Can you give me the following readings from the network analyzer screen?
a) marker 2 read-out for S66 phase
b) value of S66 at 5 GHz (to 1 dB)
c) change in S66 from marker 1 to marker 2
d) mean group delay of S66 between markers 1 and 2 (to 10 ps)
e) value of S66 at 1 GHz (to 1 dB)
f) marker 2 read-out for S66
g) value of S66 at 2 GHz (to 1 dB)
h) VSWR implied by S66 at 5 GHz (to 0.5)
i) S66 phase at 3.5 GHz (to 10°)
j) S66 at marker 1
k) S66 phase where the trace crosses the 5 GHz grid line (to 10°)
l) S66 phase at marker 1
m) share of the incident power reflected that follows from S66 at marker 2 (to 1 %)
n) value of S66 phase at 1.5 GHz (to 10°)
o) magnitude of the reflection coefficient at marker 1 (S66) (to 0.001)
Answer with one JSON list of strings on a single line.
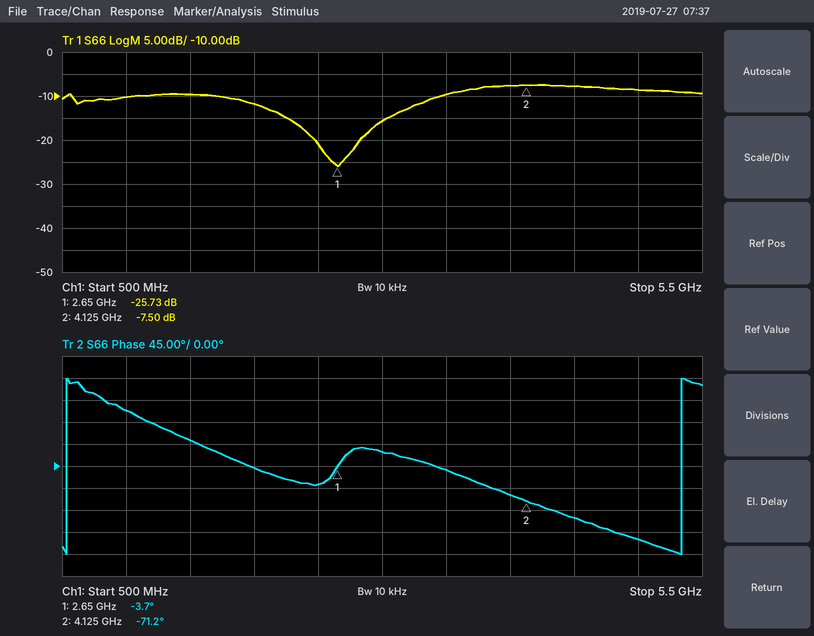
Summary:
["-71.2°", "-9 dB", "18.23 dB", "130 ps", "-10 dB", "-7.50 dB", "-12 dB", "2.0", "-10°", "-25.73 dB", "-150°", "-3.7°", "18 %", "50°", "0.052"]
